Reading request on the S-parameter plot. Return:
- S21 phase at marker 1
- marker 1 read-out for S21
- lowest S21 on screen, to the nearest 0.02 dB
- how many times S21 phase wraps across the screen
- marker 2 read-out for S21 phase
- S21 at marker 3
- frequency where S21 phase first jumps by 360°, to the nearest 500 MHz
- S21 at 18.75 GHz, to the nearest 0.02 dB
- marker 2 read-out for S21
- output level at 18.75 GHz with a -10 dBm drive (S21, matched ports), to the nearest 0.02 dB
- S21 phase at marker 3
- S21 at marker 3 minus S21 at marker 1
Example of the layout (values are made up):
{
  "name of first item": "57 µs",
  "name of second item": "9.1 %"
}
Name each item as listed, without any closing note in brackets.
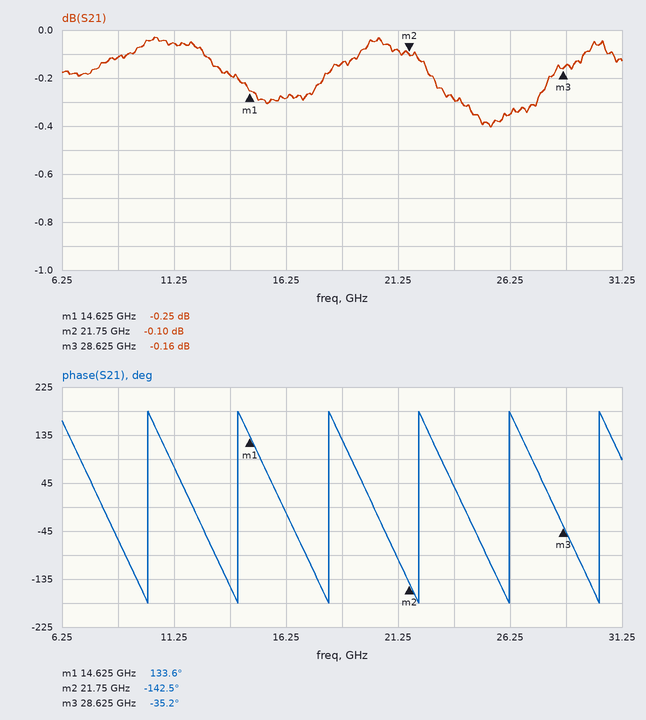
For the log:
{
  "S21 phase at marker 1": "133.6°",
  "marker 1 read-out for S21": "-0.25 dB",
  "lowest S21 on screen, to the nearest 0.02 dB": "-0.40 dB",
  "how many times S21 phase wraps across the screen": "6",
  "marker 2 read-out for S21 phase": "-142.5°",
  "S21 at marker 3": "-0.16 dB",
  "frequency where S21 phase first jumps by 360°, to the nearest 500 MHz": "10.0 GHz",
  "S21 at 18.75 GHz, to the nearest 0.02 dB": "-0.14 dB",
  "marker 2 read-out for S21": "-0.10 dB",
  "output level at 18.75 GHz with a -10 dBm drive (S21, matched ports), to the nearest 0.02 dB": "-10.14 dBm",
  "S21 phase at marker 3": "-35.2°",
  "S21 at marker 3 minus S21 at marker 1": "0.09 dB"
}
